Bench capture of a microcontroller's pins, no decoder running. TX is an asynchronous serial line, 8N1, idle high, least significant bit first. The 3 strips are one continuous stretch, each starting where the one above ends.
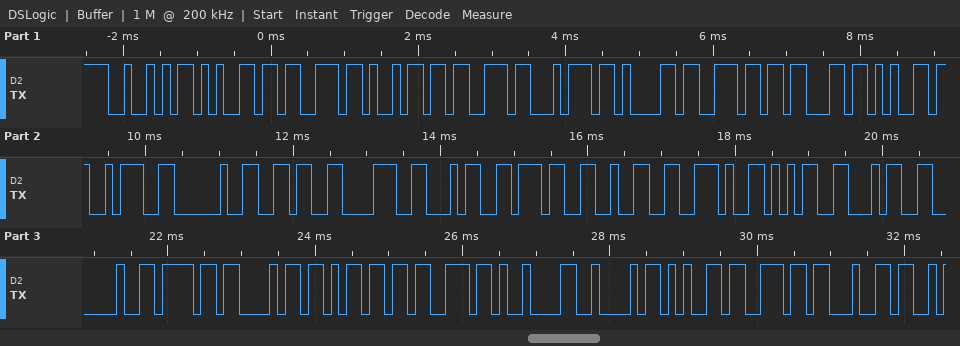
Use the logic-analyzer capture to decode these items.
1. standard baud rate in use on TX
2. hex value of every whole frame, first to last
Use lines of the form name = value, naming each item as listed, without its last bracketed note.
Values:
standard baud rate in use on TX = 9600 baud
hex value of every whole frame, first to last = 0x52 0x65 0x73 0x69 0x73 0x74 0x61 0x6E 0x63 0x65 0x3A 0x20 0x36 0x38 0x34 0x37 0x32 0x2E 0x35 0x34 0x20 0x6F 0x68 0x6D 0x73 0x09 0x42 0x65 0x6E 0x64
